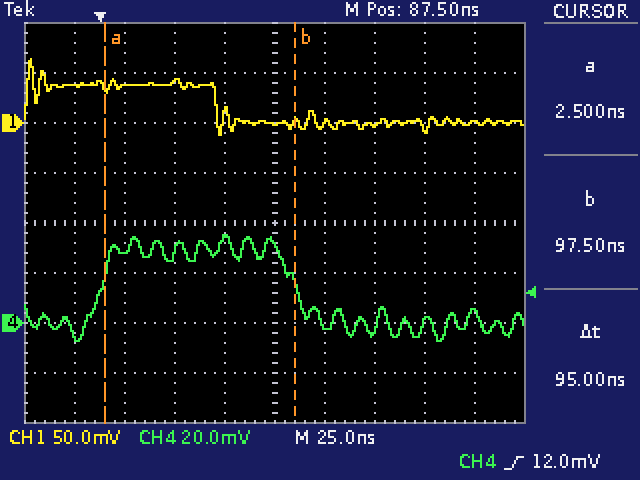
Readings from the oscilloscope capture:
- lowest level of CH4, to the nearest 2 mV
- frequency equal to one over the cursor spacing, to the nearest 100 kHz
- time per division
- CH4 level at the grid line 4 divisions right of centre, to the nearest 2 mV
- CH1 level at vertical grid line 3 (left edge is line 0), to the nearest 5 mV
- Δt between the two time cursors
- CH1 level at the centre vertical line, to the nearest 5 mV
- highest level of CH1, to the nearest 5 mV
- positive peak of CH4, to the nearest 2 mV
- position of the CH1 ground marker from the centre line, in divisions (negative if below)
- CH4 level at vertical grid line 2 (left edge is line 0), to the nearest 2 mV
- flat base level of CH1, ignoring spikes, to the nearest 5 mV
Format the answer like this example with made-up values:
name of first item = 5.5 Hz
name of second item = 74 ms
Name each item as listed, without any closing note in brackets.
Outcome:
lowest level of CH4, to the nearest 2 mV = -8 mV
frequency equal to one over the cursor spacing, to the nearest 100 kHz = 10.5 MHz
time per division = 25 ns
CH4 level at the grid line 4 divisions right of centre, to the nearest 2 mV = 4 mV
CH1 level at vertical grid line 3 (left edge is line 0), to the nearest 5 mV = 40 mV
Δt between the two time cursors = 95 ns
CH1 level at the centre vertical line, to the nearest 5 mV = 0 mV
highest level of CH1, to the nearest 5 mV = 65 mV
positive peak of CH4, to the nearest 2 mV = 36 mV
position of the CH1 ground marker from the centre line, in divisions = +2.0 div
CH4 level at vertical grid line 2 (left edge is line 0), to the nearest 2 mV = 28 mV
flat base level of CH1, ignoring spikes, to the nearest 5 mV = 0 mV
